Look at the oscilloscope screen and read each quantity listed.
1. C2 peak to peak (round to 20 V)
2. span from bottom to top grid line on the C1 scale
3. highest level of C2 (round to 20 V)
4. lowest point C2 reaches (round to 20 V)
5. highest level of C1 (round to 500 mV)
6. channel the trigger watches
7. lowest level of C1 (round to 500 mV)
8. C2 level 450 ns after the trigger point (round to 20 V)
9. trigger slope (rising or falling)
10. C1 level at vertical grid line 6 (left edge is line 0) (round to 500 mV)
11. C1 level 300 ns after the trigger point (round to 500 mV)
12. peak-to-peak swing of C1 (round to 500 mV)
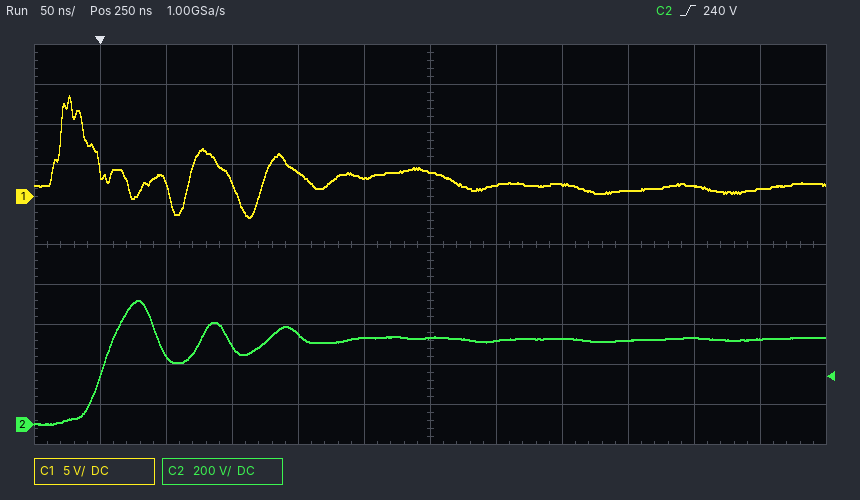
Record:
620 V
50 V
620 V
0 V
12.5 V
C2
-2.5 V
440 V
rising
3.0 V
1.5 V
15.0 V
